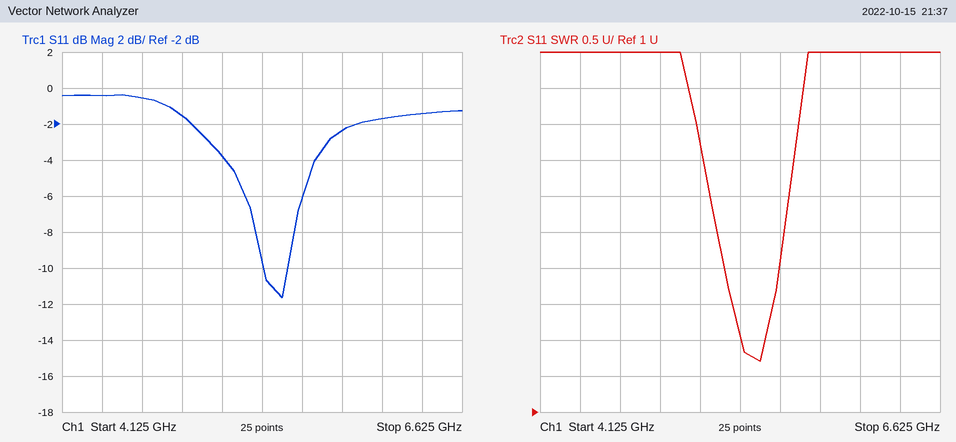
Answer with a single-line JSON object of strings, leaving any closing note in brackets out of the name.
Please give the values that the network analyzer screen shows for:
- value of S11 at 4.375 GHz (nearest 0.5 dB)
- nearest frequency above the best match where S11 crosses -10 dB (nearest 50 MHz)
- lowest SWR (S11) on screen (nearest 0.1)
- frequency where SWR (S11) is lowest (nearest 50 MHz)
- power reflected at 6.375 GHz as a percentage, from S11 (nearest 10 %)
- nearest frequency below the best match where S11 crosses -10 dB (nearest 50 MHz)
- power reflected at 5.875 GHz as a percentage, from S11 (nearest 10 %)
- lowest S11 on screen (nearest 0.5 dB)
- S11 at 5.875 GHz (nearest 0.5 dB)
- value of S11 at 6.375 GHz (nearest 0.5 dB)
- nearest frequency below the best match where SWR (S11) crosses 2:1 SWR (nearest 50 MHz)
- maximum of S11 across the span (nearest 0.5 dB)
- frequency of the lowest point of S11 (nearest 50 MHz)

{"value of S11 at 4.375 GHz": "-0.5 dB", "nearest frequency above the best match where S11 crosses -10 dB": "5.55 GHz", "lowest SWR (S11) on screen": "1.7", "frequency where SWR (S11) is lowest": "5.50 GHz", "power reflected at 6.375 GHz as a percentage, from S11": "70 %", "nearest frequency below the best match where S11 crosses -10 dB": "5.40 GHz", "power reflected at 5.875 GHz as a percentage, from S11": "60 %", "lowest S11 on screen": "-11.5 dB", "S11 at 5.875 GHz": "-2.5 dB", "value of S11 at 6.375 GHz": "-1.5 dB", "nearest frequency below the best match where SWR (S11) crosses 2:1 SWR": "5.40 GHz", "maximum of S11 across the span": "-0.5 dB", "frequency of the lowest point of S11": "5.50 GHz"}
